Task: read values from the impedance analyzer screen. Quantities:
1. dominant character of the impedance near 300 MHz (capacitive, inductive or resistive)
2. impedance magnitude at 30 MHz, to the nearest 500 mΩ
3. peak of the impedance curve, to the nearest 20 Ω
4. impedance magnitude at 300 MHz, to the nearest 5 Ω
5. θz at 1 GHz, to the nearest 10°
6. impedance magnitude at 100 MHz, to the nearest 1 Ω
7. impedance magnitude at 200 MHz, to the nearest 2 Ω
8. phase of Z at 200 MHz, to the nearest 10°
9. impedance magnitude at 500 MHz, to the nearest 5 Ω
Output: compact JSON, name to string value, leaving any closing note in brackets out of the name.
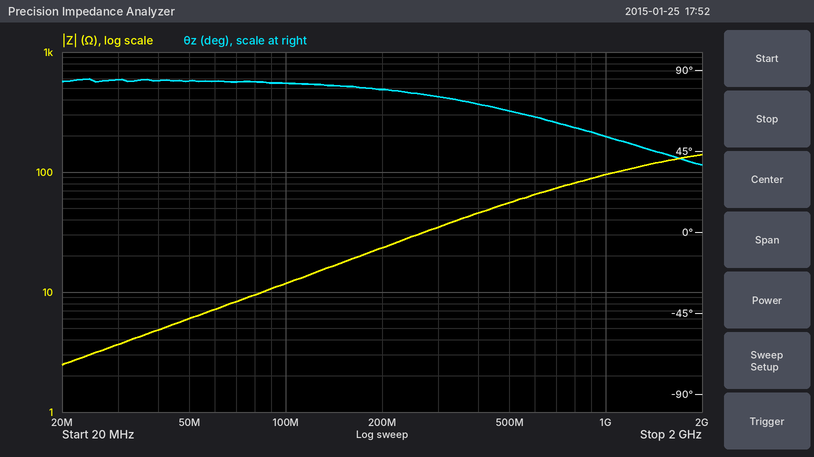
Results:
{"dominant character of the impedance near 300 MHz": "inductive", "impedance magnitude at 30 MHz, to the nearest 500 mΩ": "3.5 Ω", "peak of the impedance curve, to the nearest 20 Ω": "140 Ω", "impedance magnitude at 300 MHz, to the nearest 5 Ω": "35 Ω", "θz at 1 GHz, to the nearest 10°": "50°", "impedance magnitude at 100 MHz, to the nearest 1 Ω": "12 Ω", "impedance magnitude at 200 MHz, to the nearest 2 Ω": "24 Ω", "phase of Z at 200 MHz, to the nearest 10°": "80°", "impedance magnitude at 500 MHz, to the nearest 5 Ω": "55 Ω"}
